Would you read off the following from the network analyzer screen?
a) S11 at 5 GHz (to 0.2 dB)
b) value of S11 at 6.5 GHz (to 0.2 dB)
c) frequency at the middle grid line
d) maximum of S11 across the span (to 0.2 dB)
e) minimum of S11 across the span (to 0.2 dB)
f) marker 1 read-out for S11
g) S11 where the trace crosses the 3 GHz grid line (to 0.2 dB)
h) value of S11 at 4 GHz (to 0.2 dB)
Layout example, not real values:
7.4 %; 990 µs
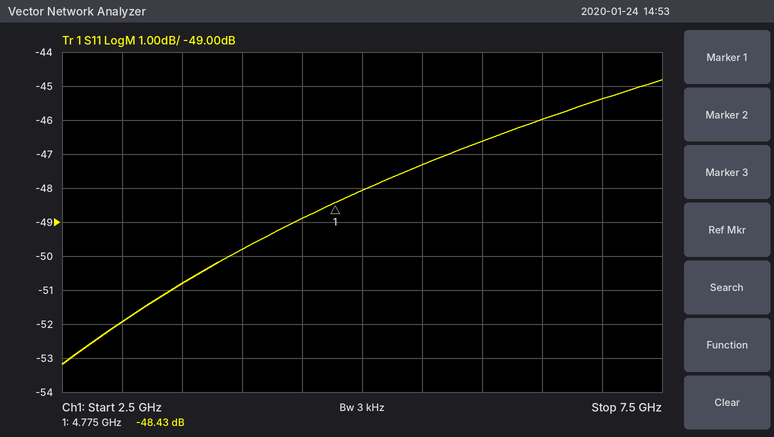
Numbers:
-48.0 dB; -46.0 dB; 5 GHz; -44.8 dB; -53.2 dB; -48.43 dB; -52.0 dB; -49.8 dB
